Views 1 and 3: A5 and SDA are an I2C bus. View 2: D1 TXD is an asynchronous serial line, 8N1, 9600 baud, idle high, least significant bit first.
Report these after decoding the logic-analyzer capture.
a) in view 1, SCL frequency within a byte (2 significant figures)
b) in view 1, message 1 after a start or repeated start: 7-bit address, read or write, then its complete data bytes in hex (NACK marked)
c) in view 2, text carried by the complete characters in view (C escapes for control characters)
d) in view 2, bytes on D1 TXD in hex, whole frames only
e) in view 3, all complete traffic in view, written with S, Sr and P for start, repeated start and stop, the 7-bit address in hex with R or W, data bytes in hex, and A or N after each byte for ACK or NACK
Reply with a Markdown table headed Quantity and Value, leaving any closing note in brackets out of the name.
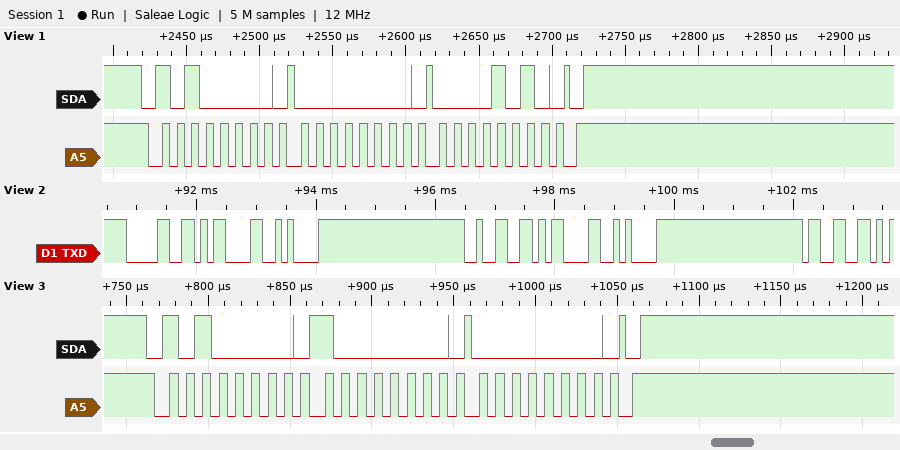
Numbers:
| Quantity | Value |
|---|---|
| in view 1, SCL frequency within a byte | 100 kHz |
| in view 1, message 1 after a start or repeated start: 7-bit address, read or write, then its complete data bytes in hex | 0x50 write: 00 0A |
| in view 2, text carried by the complete characters in view | "0\r\n2\r\n3" |
| in view 2, bytes on D1 TXD in hex, whole frames only | 30 0D 0A 32 0D 0A 33 |
| in view 3, all complete traffic in view, written with S, Sr and P for start, repeated start and stop, the 7-bit address in hex with R or W, data bytes in hex, and A or N after each byte for ACK or NACK | S 50W A 80 A 00 A P |
